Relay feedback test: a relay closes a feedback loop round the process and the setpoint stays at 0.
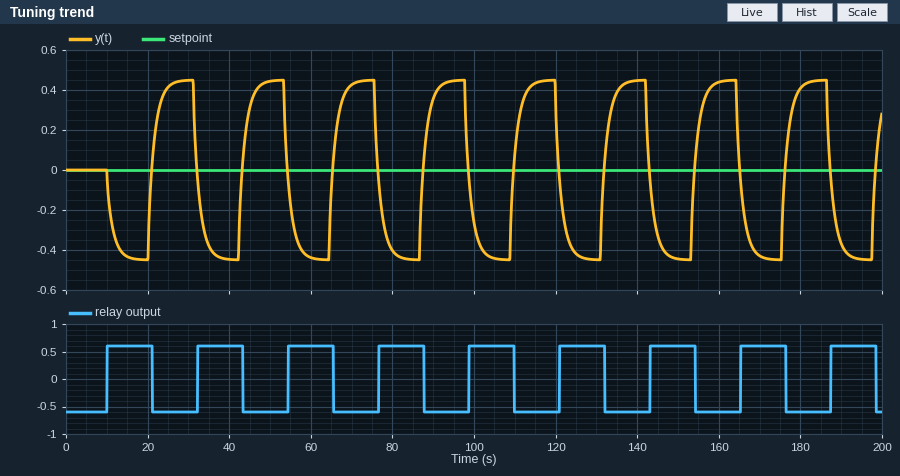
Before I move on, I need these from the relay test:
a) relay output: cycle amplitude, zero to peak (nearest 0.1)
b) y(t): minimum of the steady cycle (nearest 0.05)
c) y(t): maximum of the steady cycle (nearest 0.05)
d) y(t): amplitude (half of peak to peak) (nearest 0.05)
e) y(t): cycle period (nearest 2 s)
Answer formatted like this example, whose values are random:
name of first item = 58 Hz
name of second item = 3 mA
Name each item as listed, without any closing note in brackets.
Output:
relay output: cycle amplitude, zero to peak = 0.6
y(t): minimum of the steady cycle = -0.45
y(t): maximum of the steady cycle = 0.45
y(t): amplitude (half of peak to peak) = 0.45
y(t): cycle period = 22 s
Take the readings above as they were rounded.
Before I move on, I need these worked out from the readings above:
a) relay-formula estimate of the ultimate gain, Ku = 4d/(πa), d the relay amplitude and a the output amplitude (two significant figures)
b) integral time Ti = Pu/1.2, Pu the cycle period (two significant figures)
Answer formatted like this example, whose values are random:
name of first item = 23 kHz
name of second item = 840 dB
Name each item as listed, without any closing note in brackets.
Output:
relay-formula estimate of the ultimate gain, Ku = 4d/(πa), d the relay amplitude and a the output amplitude = 1.7
integral time Ti = Pu/1.2, Pu the cycle period = 18 s
